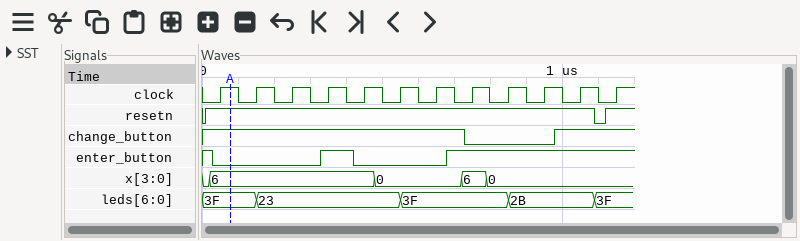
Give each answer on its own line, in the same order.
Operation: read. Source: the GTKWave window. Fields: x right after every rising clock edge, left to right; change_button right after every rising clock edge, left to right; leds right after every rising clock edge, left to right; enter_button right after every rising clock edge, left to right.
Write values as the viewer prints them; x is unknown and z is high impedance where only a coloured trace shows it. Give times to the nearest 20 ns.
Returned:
6, 6, 6, 6, 6, 0, 0, 6, 0, 0, 0, 0
1 1 1 1 1 1 1 0 0 0 1 1
3F, 23, 23, 23, 23, 3F, 3F, 3F, 2B, 2B, 2B, 3F
0 0 0 1 0 0 0 1 1 1 1 1
